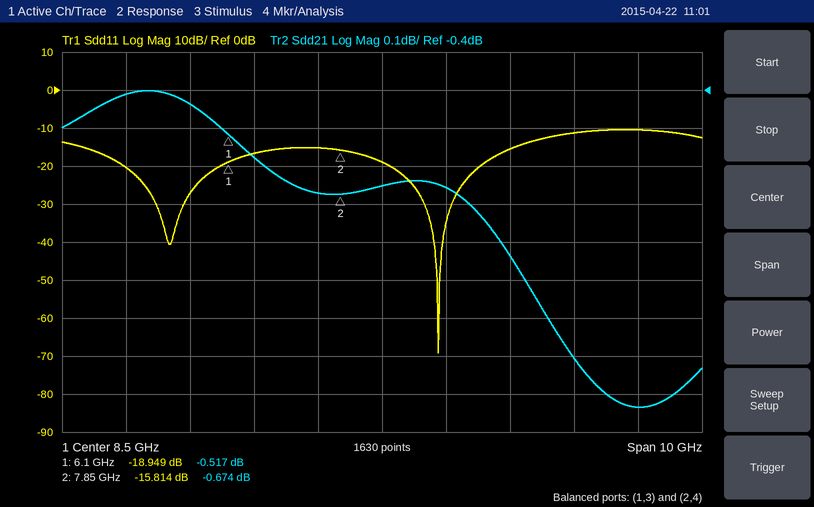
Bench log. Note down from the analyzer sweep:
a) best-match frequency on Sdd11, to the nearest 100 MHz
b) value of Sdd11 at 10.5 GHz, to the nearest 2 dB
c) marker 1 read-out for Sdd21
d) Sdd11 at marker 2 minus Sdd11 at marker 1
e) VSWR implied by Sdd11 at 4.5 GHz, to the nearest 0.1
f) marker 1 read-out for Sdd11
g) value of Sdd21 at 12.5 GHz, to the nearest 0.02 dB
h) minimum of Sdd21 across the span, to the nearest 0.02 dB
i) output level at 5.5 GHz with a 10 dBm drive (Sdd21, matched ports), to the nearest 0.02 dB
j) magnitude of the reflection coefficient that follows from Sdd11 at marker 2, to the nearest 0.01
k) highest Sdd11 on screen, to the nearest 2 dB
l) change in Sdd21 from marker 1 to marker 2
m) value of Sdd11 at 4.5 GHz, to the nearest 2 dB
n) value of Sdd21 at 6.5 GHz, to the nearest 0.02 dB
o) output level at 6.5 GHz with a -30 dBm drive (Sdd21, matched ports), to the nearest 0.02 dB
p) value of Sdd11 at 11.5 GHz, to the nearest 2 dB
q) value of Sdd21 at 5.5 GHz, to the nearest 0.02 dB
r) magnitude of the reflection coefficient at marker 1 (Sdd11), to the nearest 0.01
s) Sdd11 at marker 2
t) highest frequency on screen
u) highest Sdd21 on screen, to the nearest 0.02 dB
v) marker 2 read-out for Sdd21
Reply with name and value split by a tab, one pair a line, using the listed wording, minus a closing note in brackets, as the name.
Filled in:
best-match frequency on Sdd11, to the nearest 100 MHz	9.4 GHz
value of Sdd11 at 10.5 GHz, to the nearest 2 dB	-16 dB
marker 1 read-out for Sdd21	-0.517 dB
Sdd11 at marker 2 minus Sdd11 at marker 1	3.135 dB
VSWR implied by Sdd11 at 4.5 GHz, to the nearest 0.1	1.2
marker 1 read-out for Sdd11	-18.949 dB
value of Sdd21 at 12.5 GHz, to the nearest 0.02 dB	-1.24 dB
minimum of Sdd21 across the span, to the nearest 0.02 dB	-1.24 dB
output level at 5.5 GHz with a 10 dBm drive (Sdd21, matched ports), to the nearest 0.02 dB	9.56 dBm
magnitude of the reflection coefficient that follows from Sdd11 at marker 2, to the nearest 0.01	0.16
highest Sdd11 on screen, to the nearest 2 dB	-10 dB
change in Sdd21 from marker 1 to marker 2	-0.157 dB
value of Sdd11 at 4.5 GHz, to the nearest 2 dB	-20 dB
value of Sdd21 at 6.5 GHz, to the nearest 0.02 dB	-0.58 dB
output level at 6.5 GHz with a -30 dBm drive (Sdd21, matched ports), to the nearest 0.02 dB	-30.58 dBm
value of Sdd11 at 11.5 GHz, to the nearest 2 dB	-12 dB
value of Sdd21 at 5.5 GHz, to the nearest 0.02 dB	-0.44 dB
magnitude of the reflection coefficient at marker 1 (Sdd11), to the nearest 0.01	0.11
Sdd11 at marker 2	-15.814 dB
highest frequency on screen	13.5 GHz
highest Sdd21 on screen, to the nearest 0.02 dB	-0.40 dB
marker 2 read-out for Sdd21	-0.674 dB
